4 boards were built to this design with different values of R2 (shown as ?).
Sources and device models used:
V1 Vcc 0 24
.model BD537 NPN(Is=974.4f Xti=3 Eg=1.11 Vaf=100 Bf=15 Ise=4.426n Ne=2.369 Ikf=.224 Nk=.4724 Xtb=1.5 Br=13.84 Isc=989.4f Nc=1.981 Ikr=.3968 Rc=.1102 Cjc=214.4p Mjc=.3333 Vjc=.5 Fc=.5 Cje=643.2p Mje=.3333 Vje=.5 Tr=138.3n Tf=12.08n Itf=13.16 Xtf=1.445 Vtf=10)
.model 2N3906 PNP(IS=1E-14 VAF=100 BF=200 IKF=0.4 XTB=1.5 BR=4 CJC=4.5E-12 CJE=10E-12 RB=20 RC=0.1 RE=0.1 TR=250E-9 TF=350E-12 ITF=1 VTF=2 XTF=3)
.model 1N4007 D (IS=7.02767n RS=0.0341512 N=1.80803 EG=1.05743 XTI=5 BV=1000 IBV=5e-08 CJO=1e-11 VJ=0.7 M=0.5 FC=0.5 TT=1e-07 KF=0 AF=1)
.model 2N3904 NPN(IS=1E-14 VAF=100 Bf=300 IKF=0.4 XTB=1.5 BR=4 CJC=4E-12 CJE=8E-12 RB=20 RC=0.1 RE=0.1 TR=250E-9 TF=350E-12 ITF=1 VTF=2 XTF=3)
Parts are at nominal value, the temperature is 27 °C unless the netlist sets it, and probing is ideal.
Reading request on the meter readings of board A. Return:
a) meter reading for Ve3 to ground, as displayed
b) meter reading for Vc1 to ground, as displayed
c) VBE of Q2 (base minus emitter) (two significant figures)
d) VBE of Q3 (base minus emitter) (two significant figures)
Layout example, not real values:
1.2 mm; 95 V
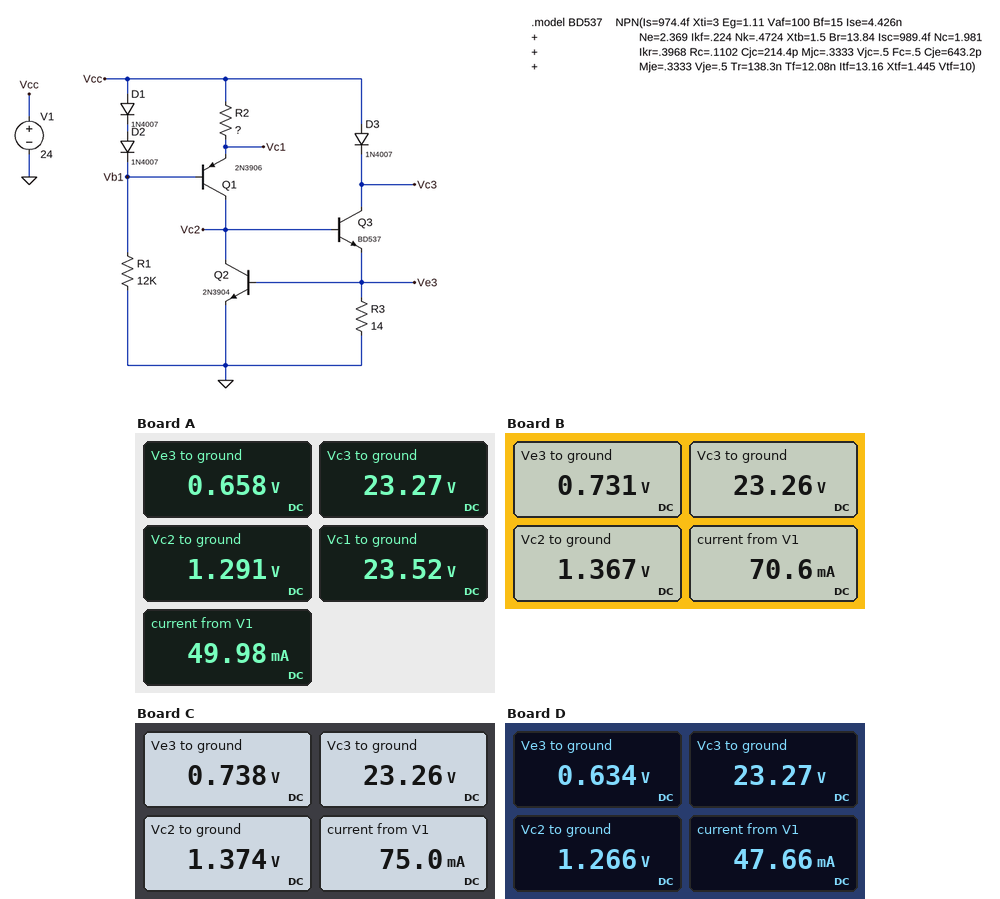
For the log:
0.658 V; 23.52 V; 660 mV; 630 mV
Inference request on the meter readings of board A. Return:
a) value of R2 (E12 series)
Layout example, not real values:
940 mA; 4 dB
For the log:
120 Ω
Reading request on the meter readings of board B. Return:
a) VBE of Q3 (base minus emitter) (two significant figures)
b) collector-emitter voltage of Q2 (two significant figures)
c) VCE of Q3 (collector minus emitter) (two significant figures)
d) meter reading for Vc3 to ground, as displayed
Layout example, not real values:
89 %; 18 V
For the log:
640 mV; 1.4 V; 23 V; 23.26 V
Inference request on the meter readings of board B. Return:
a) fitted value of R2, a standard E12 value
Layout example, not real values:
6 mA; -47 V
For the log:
22 Ω
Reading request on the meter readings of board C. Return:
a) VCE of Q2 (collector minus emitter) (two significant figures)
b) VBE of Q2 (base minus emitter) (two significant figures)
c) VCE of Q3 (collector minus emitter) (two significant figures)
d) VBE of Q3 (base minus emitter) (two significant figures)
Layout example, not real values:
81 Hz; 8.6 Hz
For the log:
1.4 V; 740 mV; 23 V; 640 mV
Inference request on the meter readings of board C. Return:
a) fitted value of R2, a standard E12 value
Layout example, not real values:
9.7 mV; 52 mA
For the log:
18 Ω
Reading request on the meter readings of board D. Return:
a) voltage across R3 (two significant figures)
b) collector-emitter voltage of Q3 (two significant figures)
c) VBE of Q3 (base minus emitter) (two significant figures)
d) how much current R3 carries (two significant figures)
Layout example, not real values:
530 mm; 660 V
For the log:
630 mV; 23 V; 630 mV; 45 mA
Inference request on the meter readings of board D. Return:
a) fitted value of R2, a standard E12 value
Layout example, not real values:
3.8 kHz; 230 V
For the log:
150 Ω
